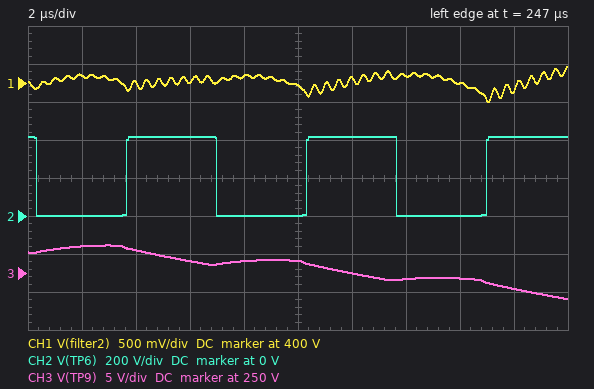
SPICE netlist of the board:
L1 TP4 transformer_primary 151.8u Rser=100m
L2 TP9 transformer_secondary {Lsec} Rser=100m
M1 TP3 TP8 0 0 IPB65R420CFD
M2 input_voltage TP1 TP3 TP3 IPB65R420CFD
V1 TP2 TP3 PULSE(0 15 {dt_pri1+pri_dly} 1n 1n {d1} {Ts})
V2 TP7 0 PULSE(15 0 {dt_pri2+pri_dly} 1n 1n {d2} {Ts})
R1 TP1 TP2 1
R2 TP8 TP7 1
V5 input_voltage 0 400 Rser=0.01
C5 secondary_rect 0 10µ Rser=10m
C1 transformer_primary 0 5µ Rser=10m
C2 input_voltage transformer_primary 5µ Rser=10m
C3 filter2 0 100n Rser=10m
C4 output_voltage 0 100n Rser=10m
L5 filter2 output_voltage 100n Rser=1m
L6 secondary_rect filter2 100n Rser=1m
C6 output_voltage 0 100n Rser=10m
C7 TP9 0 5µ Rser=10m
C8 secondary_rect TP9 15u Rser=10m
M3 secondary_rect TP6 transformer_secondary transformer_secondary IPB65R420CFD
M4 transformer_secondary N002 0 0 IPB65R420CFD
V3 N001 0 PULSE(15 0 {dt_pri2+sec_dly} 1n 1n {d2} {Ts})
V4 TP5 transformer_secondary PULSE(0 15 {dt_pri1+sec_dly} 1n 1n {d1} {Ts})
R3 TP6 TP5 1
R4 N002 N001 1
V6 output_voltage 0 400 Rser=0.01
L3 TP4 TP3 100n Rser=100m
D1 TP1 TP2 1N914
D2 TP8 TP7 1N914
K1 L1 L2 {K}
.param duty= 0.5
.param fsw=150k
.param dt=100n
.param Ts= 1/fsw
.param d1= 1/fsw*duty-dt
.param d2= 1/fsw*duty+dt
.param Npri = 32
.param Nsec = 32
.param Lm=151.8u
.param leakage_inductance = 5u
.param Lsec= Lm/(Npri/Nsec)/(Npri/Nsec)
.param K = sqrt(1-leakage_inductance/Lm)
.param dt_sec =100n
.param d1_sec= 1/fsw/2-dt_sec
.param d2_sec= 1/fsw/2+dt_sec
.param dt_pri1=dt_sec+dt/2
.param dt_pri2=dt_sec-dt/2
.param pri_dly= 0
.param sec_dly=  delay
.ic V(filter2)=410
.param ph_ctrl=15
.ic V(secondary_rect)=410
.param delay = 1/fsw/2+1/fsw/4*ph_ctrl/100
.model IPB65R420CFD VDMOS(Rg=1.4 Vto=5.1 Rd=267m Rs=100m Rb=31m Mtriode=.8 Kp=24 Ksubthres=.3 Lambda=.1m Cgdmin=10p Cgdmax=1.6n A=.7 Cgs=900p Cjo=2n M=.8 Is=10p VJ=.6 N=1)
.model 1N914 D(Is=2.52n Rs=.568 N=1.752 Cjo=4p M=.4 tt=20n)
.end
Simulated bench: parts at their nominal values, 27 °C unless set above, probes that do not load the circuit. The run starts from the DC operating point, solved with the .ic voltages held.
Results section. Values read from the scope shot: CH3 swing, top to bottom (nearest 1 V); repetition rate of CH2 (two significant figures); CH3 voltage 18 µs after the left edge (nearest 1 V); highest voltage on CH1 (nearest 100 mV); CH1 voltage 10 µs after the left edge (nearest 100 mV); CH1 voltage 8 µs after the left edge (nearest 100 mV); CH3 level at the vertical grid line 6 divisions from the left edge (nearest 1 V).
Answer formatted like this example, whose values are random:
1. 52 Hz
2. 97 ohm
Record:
1. 7 V
2. 150 kHz
3. 248 V
4. 400.2 V
5. 400.0 V
6. 400.1 V
7. 250 V
